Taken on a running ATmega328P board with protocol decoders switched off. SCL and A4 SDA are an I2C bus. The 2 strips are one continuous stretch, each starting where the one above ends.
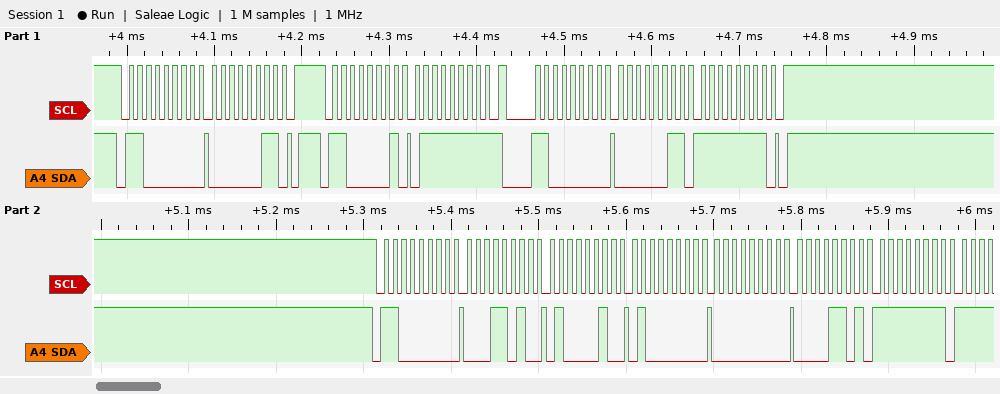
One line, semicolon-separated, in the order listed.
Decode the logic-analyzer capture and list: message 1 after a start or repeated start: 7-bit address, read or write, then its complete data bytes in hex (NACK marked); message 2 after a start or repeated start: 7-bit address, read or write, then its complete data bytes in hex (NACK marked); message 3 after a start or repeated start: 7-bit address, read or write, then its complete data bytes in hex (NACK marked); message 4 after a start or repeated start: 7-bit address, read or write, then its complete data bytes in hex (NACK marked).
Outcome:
0x60 write: 03; 0x60 read: 7F NACK; 0x60 write: 03 FF; 0x60 write: 1A 42 40 00 0D FF
